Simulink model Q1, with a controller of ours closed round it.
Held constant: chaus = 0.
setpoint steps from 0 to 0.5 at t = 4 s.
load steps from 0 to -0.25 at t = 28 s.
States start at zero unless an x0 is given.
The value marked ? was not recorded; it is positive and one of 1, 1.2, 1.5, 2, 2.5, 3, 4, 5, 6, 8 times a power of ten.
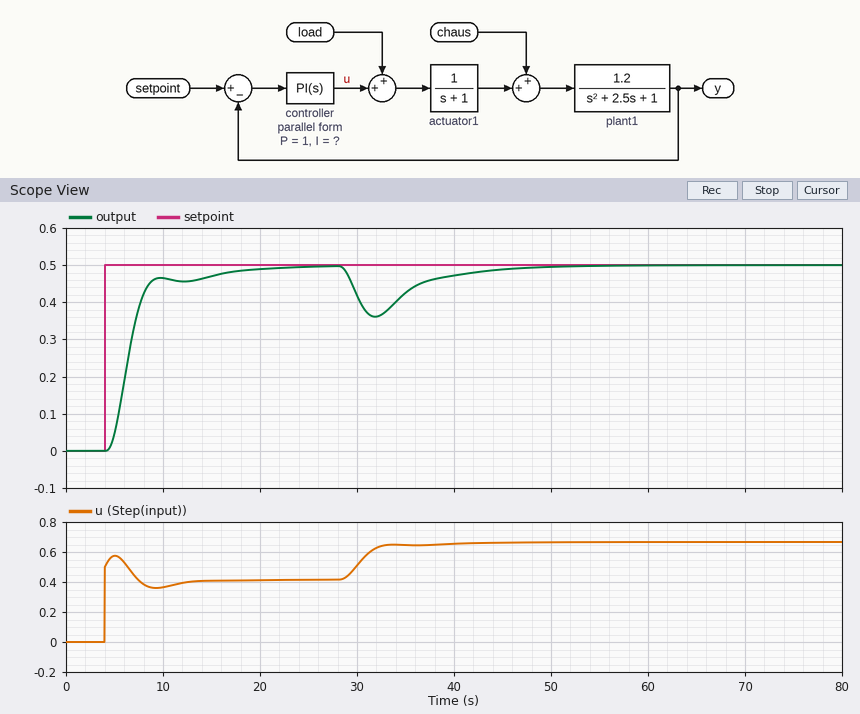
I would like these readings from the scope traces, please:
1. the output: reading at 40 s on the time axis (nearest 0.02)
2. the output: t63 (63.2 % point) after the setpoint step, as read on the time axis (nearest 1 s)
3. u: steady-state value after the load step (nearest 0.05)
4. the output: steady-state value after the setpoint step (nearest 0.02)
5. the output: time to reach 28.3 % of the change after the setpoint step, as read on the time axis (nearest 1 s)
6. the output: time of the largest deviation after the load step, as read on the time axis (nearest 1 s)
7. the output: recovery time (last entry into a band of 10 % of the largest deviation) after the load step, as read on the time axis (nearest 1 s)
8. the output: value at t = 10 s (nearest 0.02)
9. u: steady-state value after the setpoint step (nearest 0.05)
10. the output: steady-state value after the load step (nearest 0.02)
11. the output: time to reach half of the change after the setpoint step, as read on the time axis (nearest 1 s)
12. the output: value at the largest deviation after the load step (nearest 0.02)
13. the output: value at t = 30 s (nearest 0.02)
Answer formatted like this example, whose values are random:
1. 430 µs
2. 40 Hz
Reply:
1. 0.48
2. 7 s
3. 0.65
4. 0.50
5. 6 s
6. 32 s
7. 44 s
8. 0.46
9. 0.40
10. 0.50
11. 6 s
12. 0.36
13. 0.42
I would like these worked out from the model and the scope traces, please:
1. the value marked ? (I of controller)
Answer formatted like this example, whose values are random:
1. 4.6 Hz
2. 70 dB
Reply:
1. 0.25
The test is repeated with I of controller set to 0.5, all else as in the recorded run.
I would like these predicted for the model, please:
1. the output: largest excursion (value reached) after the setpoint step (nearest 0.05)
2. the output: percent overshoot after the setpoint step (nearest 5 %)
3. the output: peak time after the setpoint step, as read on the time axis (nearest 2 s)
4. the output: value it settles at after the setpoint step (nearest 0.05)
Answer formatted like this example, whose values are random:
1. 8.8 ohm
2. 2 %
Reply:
1. 0.60
2. 20 %
3. 10 s
4. 0.50
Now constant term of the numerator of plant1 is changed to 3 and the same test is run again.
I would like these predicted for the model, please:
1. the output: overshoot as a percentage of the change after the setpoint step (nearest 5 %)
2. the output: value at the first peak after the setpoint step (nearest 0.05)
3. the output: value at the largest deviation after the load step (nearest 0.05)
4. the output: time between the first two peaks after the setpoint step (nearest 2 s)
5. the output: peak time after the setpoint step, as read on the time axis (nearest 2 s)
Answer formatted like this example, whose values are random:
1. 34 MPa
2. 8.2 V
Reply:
1. 30 %
2. 0.65
3. 0.25
4. 6 s
5. 8 s
